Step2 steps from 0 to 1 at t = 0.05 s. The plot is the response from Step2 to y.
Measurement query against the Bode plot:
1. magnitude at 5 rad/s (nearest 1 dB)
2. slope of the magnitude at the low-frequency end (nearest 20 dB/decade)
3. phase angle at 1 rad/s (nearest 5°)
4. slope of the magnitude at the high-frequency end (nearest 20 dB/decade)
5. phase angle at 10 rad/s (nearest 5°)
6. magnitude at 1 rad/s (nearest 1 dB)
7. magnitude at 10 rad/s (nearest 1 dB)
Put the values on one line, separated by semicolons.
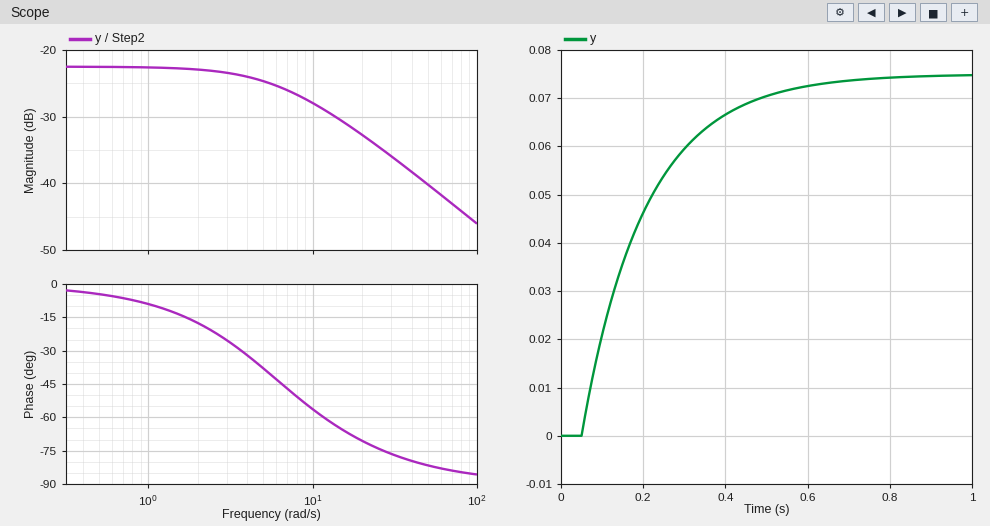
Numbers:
-25 dB; 0 dB/decade; -10°; -20 dB/decade; -55°; -23 dB; -28 dB
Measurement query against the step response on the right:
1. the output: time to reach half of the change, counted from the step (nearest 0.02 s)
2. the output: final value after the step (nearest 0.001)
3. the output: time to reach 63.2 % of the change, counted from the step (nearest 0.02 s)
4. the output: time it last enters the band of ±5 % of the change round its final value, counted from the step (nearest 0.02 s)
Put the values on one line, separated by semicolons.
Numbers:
0.10 s; 0.075; 0.16 s; 0.48 s
